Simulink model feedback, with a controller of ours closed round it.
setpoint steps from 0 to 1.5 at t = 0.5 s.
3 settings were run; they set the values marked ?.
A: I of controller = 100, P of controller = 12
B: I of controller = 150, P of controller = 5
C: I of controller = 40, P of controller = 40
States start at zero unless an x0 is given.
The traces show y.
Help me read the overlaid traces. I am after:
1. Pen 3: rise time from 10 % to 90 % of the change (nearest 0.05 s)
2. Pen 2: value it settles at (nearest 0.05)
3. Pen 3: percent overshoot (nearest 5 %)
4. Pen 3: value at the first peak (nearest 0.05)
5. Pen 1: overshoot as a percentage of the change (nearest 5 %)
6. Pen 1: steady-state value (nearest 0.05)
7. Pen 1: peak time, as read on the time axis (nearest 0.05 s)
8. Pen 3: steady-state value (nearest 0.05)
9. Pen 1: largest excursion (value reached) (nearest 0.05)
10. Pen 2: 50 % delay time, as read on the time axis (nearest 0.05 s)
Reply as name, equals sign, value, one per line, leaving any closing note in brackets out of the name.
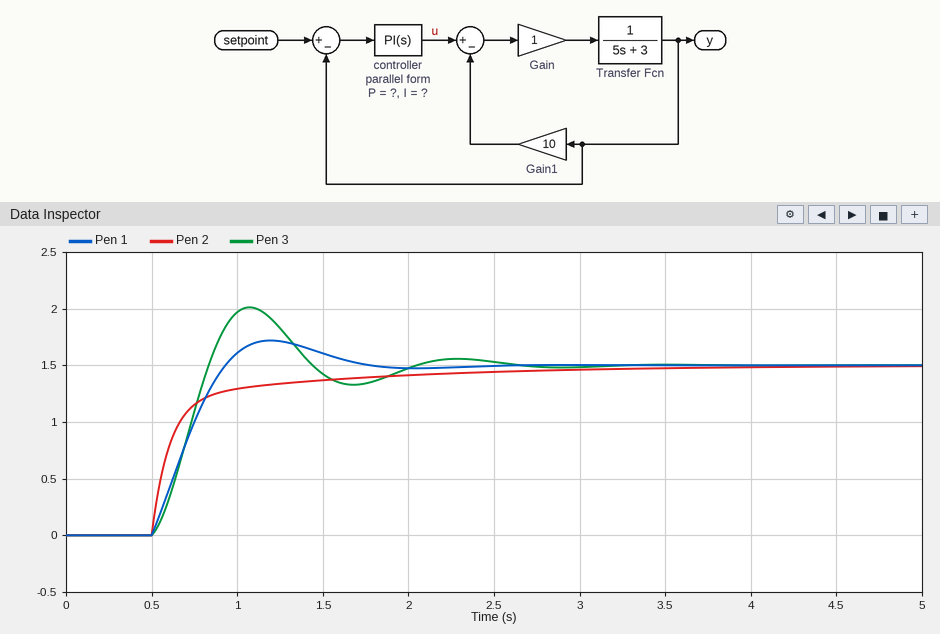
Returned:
Pen 3: rise time from 10 % to 90 % of the change = 0.25 s
Pen 2: value it settles at = 1.50
Pen 3: percent overshoot = 35 %
Pen 3: value at the first peak = 2.00
Pen 1: overshoot as a percentage of the change = 15 %
Pen 1: steady-state value = 1.50
Pen 1: peak time, as read on the time axis = 1.20 s
Pen 3: steady-state value = 1.50
Pen 1: largest excursion (value reached) = 1.70
Pen 2: 50 % delay time, as read on the time axis = 0.60 s
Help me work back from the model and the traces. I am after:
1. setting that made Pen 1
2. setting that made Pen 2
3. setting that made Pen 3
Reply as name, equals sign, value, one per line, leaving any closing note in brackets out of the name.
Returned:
setting that made Pen 1 = A
setting that made Pen 2 = C
setting that made Pen 3 = B
